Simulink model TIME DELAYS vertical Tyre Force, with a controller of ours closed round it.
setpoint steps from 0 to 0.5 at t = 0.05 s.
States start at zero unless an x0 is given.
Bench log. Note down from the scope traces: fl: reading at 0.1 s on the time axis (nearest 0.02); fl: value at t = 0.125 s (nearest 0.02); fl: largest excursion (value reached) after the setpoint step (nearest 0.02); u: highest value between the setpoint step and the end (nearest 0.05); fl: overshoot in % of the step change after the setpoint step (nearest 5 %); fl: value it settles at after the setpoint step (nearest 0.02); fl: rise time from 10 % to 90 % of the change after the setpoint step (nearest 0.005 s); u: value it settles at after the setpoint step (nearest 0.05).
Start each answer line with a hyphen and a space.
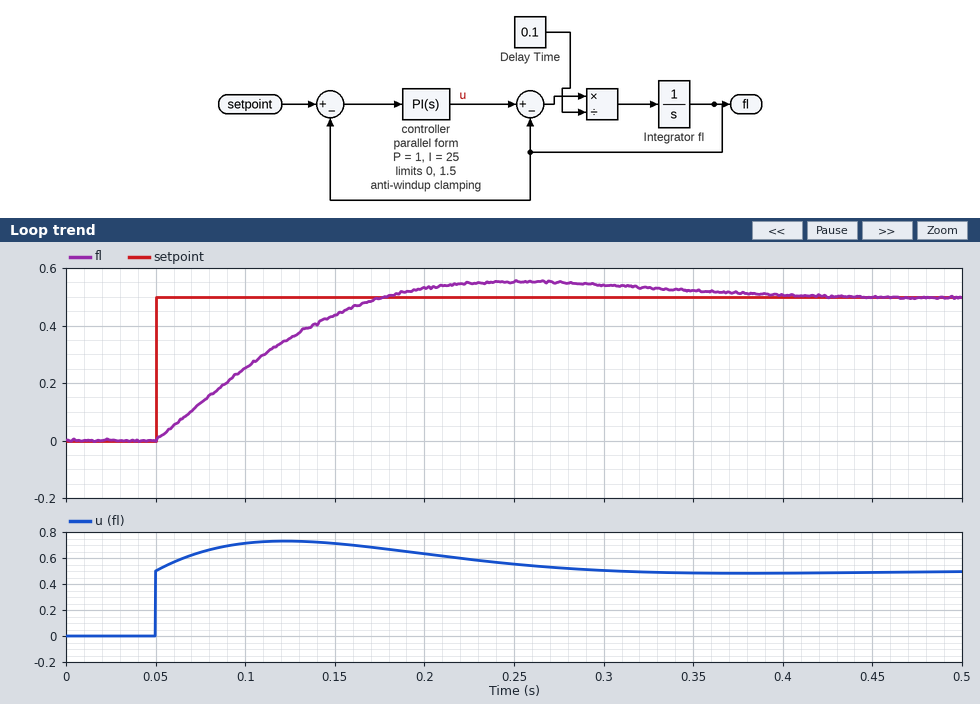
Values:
- 0.26
- 0.36
- 0.56
- 0.75
- 10 %
- 0.50
- 0.095 s
- 0.50
